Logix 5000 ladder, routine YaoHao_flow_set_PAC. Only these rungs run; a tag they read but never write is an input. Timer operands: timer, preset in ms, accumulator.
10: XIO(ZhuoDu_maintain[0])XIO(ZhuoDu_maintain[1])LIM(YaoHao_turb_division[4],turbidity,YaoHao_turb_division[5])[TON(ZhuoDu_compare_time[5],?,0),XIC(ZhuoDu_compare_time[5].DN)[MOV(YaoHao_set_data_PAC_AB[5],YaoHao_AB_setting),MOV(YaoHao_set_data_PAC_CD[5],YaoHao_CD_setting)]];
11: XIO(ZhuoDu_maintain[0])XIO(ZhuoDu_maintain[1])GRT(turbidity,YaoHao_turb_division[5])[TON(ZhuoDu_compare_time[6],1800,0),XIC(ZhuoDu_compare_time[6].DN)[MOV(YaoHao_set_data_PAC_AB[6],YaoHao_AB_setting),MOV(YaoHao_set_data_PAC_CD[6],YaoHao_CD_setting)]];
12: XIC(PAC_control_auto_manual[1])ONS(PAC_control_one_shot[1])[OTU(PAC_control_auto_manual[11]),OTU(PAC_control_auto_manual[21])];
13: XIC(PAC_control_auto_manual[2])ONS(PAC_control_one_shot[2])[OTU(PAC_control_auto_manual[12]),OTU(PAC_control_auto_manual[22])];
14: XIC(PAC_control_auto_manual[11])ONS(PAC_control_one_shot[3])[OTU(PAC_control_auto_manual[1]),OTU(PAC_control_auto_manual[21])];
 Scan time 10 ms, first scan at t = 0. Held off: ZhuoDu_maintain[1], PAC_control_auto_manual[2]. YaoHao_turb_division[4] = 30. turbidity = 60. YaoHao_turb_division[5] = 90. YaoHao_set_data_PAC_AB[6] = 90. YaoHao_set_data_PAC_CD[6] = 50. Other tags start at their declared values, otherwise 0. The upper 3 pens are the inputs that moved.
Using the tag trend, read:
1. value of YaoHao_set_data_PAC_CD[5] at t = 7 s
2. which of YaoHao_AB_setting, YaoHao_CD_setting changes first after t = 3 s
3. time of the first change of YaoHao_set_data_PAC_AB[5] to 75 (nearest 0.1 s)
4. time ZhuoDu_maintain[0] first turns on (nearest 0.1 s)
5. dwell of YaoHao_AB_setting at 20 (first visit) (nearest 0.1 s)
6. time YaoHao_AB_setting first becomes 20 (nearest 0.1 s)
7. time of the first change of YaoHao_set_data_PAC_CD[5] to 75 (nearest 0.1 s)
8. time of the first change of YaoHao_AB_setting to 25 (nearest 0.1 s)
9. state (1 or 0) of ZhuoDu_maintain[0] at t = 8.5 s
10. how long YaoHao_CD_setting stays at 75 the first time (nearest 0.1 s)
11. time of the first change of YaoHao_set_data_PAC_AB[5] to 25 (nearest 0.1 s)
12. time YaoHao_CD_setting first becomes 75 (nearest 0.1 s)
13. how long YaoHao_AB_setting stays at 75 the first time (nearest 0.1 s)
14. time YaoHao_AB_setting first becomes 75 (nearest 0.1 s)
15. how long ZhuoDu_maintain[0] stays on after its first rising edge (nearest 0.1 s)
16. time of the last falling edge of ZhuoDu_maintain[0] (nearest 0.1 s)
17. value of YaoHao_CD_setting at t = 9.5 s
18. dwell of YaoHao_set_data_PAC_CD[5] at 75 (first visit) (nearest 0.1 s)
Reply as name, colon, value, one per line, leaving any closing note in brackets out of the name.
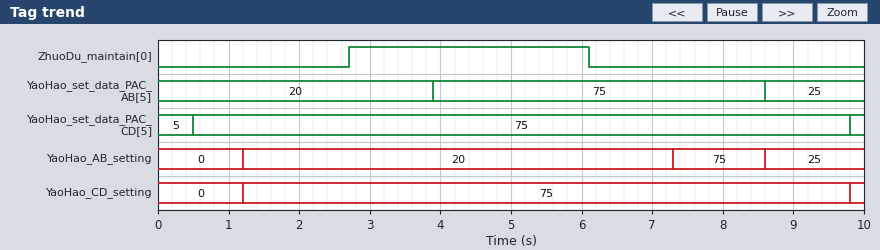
value of YaoHao_set_data_PAC_CD[5] at t = 7 s: 75
which of YaoHao_AB_setting, YaoHao_CD_setting changes first after t = 3 s: YaoHao_AB_setting
time of the first change of YaoHao_set_data_PAC_AB[5] to 75: 3.9 s
time ZhuoDu_maintain[0] first turns on: 2.7 s
dwell of YaoHao_AB_setting at 20 (first visit): 6.1 s
time YaoHao_AB_setting first becomes 20: 1.2 s
time of the first change of YaoHao_set_data_PAC_CD[5] to 75: 0.5 s
time of the first change of YaoHao_AB_setting to 25: 8.6 s
state (1 or 0) of ZhuoDu_maintain[0] at t = 8.5 s: 0
how long YaoHao_CD_setting stays at 75 the first time: 8.6 s
time of the first change of YaoHao_set_data_PAC_AB[5] to 25: 8.6 s
time YaoHao_CD_setting first becomes 75: 1.2 s
how long YaoHao_AB_setting stays at 75 the first time: 1.3 s
time YaoHao_AB_setting first becomes 75: 7.3 s
how long ZhuoDu_maintain[0] stays on after its first rising edge: 3.4 s
time of the last falling edge of ZhuoDu_maintain[0]: 6.1 s
value of YaoHao_CD_setting at t = 9.5 s: 75
dwell of YaoHao_set_data_PAC_CD[5] at 75 (first visit): 9.3 s
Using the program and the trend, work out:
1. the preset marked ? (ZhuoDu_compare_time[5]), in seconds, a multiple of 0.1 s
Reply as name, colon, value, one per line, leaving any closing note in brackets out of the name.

the preset marked ? (ZhuoDu_compare_time[5]), in seconds, a multiple of 0.1 s: 1.2 s
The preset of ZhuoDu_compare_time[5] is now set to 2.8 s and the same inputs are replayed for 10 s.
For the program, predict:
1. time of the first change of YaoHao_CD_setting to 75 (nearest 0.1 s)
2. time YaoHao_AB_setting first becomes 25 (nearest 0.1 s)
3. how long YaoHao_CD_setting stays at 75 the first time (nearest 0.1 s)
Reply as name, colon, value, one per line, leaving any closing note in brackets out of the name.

time of the first change of YaoHao_CD_setting to 75: 8.9 s
time YaoHao_AB_setting first becomes 25: 8.9 s
how long YaoHao_CD_setting stays at 75 the first time: 0.9 s
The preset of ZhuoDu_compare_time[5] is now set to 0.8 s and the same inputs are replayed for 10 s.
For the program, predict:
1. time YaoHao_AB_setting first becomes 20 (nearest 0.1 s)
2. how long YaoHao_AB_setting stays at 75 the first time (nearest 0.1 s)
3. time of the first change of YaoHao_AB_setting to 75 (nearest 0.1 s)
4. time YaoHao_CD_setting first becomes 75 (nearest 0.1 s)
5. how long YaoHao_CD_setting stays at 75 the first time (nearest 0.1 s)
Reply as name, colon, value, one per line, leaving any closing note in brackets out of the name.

time YaoHao_AB_setting first becomes 20: 0.8 s
how long YaoHao_AB_setting stays at 75 the first time: 1.7 s
time of the first change of YaoHao_AB_setting to 75: 6.9 s
time YaoHao_CD_setting first becomes 75: 0.8 s
how long YaoHao_CD_setting stays at 75 the first time: 9.0 s
